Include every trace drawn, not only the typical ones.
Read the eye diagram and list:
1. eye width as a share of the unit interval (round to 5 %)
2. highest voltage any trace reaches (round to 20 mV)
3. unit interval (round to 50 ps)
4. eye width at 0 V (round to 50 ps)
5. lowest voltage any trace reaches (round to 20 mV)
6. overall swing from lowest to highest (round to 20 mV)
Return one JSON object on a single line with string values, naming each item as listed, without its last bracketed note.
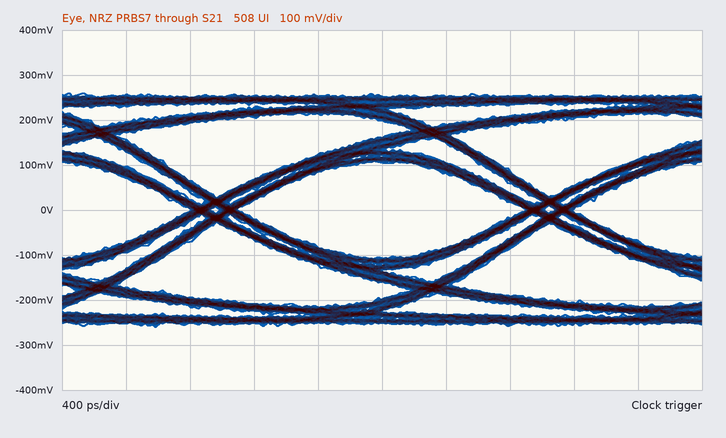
{"eye width as a share of the unit interval": "85 %", "highest voltage any trace reaches": "260 mV", "unit interval": "2.10 ns", "eye width at 0 V": "1.80 ns", "lowest voltage any trace reaches": "-260 mV", "overall swing from lowest to highest": "520 mV"}
